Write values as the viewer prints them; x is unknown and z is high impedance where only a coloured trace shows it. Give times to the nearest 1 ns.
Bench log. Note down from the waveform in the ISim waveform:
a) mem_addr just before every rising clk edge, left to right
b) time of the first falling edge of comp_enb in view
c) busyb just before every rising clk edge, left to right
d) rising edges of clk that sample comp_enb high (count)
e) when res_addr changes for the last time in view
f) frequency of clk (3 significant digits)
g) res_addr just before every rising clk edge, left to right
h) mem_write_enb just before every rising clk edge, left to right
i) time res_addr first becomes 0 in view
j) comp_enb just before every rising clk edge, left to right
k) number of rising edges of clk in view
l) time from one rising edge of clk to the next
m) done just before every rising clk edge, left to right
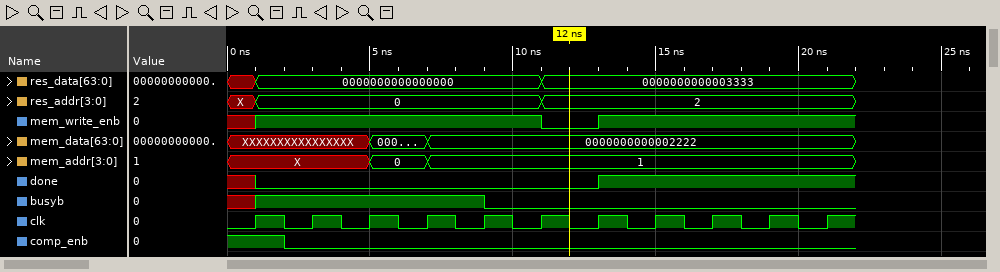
X, X, X, 0, 1, 1, 1, 1, 1, 1, 1
2 ns
x 1 1 1 1 0 0 0 0 0 0
1
11 ns
500 MHz
X, 0, 0, 0, 0, 0, 2, 2, 2, 2, 2
x 1 1 1 1 1 0 1 1 1 1
1 ns
1 0 0 0 0 0 0 0 0 0 0
11
2 ns
x 0 0 0 0 0 0 1 1 1 1
